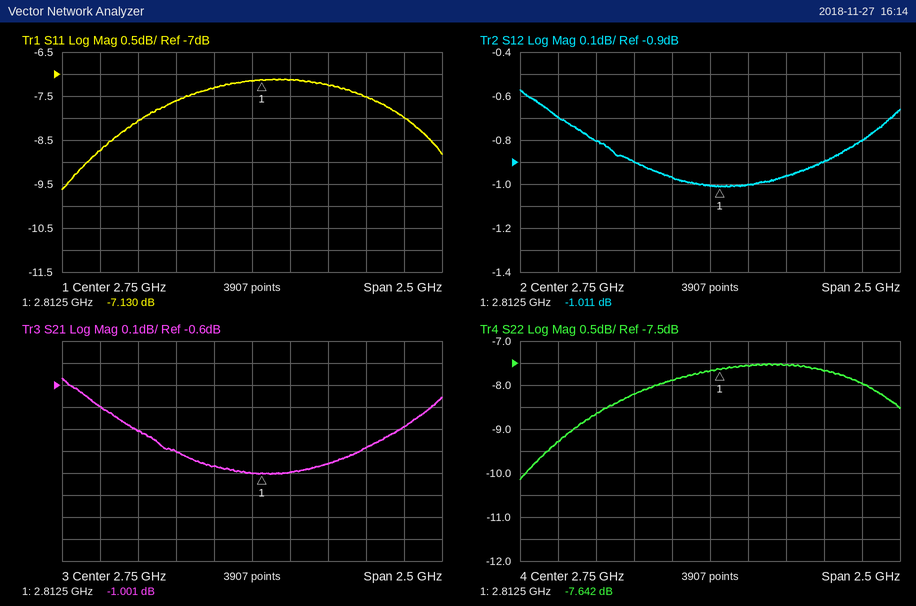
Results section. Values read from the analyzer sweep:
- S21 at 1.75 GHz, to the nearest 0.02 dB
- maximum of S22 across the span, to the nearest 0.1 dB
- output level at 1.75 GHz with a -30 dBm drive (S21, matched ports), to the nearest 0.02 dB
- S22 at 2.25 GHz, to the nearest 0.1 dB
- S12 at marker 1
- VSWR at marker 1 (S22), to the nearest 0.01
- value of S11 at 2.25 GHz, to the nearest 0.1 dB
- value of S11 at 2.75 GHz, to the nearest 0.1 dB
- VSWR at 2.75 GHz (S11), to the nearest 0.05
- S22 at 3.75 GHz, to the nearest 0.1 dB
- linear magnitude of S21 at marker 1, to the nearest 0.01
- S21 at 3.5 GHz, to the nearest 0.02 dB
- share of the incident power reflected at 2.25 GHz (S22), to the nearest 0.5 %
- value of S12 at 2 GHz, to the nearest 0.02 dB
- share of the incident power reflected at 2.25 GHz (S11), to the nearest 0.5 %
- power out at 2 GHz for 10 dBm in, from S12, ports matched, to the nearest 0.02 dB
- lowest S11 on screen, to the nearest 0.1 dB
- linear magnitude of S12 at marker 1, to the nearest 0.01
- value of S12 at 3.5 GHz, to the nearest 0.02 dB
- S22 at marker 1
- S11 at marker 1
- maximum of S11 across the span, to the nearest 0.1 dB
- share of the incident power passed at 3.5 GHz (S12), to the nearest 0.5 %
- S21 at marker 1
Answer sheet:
-0.70 dB
-7.5 dB
-30.70 dBm
-8.2 dB
-1.011 dB
2.42
-7.6 dB
-7.2 dB
2.55
-8.0 dB
0.89
-0.88 dB
15.0 %
-0.80 dB
17.5 %
9.20 dBm
-9.6 dB
0.89
-0.90 dB
-7.642 dB
-7.130 dB
-7.1 dB
81.5 %
-1.001 dB
